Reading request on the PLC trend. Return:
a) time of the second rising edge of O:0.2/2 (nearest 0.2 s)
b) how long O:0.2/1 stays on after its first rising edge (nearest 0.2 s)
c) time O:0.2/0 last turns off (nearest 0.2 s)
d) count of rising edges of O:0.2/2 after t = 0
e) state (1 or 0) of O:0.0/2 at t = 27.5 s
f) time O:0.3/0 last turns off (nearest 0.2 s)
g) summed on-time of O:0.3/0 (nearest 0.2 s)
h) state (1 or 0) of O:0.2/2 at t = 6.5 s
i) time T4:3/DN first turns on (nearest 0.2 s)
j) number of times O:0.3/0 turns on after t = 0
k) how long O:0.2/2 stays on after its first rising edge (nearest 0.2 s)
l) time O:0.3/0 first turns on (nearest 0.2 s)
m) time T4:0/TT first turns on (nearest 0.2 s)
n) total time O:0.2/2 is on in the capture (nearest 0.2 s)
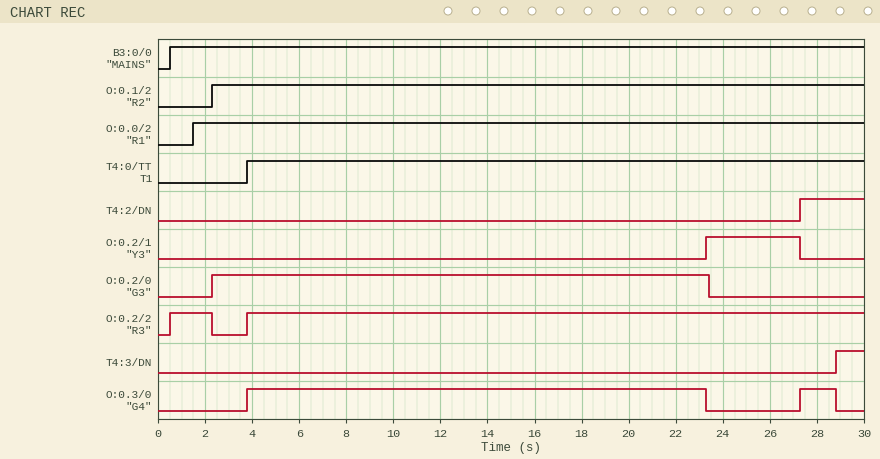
3.8 s
4.0 s
23.4 s
2
1
28.8 s
21.0 s
1
28.8 s
2
1.8 s
3.8 s
3.8 s
28.0 s
